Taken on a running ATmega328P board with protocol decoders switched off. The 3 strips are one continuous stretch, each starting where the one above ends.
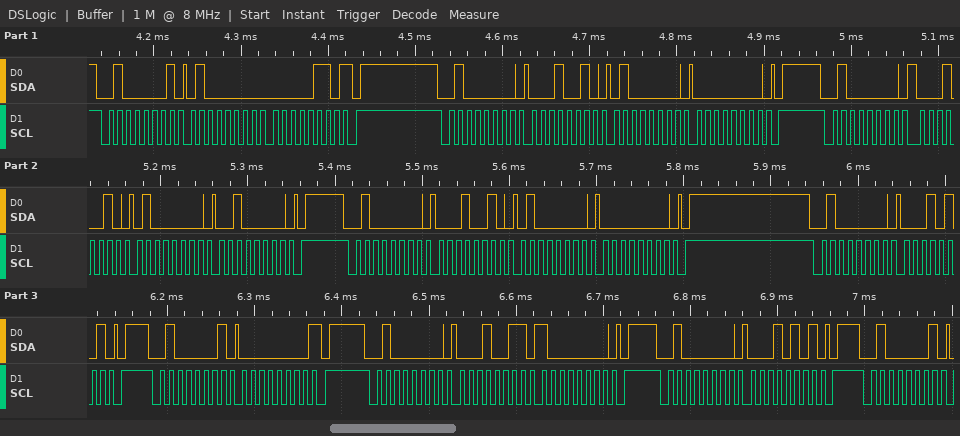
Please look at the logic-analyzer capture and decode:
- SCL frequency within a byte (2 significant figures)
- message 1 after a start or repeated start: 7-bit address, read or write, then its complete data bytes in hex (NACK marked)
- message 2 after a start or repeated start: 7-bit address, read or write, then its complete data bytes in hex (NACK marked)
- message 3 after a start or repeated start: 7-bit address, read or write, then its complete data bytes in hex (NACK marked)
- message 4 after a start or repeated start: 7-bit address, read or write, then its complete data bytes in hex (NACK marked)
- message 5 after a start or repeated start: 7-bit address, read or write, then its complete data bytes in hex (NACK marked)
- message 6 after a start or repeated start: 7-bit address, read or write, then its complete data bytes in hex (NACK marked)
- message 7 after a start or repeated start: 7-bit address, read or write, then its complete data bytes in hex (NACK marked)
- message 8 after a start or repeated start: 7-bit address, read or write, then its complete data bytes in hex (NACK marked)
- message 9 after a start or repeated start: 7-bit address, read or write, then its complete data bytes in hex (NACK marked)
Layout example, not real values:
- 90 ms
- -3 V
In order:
- 100 kHz
- 0x20 read: 40 06 NACK
- 0x20 write: 12 40 00
- 0x20 write: 12 40 20
- 0x20 write: 12 40 00
- 0x20 write: 15
- 0x20 read: 00 NACK
- 0x20 write: 13 80
- 0x20 write: 15
- 0x20 read
